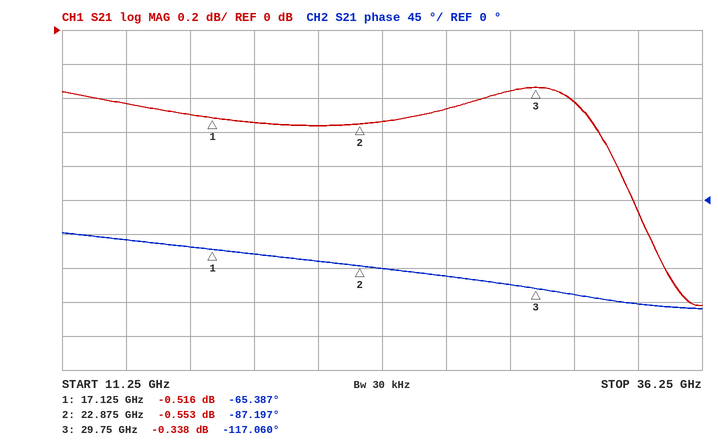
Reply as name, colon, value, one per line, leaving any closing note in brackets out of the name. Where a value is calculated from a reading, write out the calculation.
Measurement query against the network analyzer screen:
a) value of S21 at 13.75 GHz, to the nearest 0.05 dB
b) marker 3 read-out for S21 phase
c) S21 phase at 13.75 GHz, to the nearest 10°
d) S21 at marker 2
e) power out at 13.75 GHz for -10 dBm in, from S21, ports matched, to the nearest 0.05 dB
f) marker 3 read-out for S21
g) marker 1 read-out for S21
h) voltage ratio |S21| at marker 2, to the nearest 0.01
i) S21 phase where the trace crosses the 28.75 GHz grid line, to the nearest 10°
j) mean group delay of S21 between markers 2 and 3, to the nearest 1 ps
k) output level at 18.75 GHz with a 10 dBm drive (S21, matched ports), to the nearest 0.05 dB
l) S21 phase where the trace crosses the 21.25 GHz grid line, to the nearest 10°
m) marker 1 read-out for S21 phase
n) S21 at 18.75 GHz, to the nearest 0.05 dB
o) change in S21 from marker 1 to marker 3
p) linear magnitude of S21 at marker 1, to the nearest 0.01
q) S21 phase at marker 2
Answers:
value of S21 at 13.75 GHz, to the nearest 0.05 dB: -0.45 dB
marker 3 read-out for S21 phase: -117.060°
S21 phase at 13.75 GHz, to the nearest 10°: -50°
S21 at marker 2: -0.553 dB
power out at 13.75 GHz for -10 dBm in, from S21, ports matched, to the nearest 0.05 dB: -10 dBm + (-0.45 dB) = -10.45 dBm
marker 3 read-out for S21: -0.338 dB
marker 1 read-out for S21: -0.516 dB
voltage ratio |S21| at marker 2, to the nearest 0.01: 10^(-0.553/20) ≈ 0.94
S21 phase where the trace crosses the 28.75 GHz grid line, to the nearest 10°: -110°
mean group delay of S21 between markers 2 and 3, to the nearest 1 ps: −(-117.06° − (-87.197°))/(360° × 6.875 GHz) ≈ 12 ps
output level at 18.75 GHz with a 10 dBm drive (S21, matched ports), to the nearest 0.05 dB: 10 dBm + (-0.55 dB) = 9.45 dBm
S21 phase where the trace crosses the 21.25 GHz grid line, to the nearest 10°: -80°
marker 1 read-out for S21 phase: -65.387°
S21 at 18.75 GHz, to the nearest 0.05 dB: -0.55 dB
change in S21 from marker 1 to marker 3: -0.338 − (-0.516) = 0.178 dB
linear magnitude of S21 at marker 1, to the nearest 0.01: 10^(-0.516/20) ≈ 0.94
S21 phase at marker 2: -87.197°
